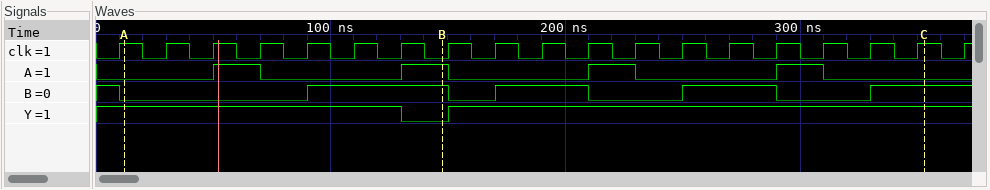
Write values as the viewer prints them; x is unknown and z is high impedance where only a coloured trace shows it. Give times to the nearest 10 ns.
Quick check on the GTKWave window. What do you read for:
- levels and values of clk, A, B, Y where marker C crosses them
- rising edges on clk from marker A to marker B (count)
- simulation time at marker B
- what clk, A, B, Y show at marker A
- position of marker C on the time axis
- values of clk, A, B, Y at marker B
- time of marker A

clk=1, A=0, B=1, Y=1
6
150 ns
clk=1, A=0, B=0, Y=1
350 ns
clk=0, A=1, B=1, Y=0
10 ns
